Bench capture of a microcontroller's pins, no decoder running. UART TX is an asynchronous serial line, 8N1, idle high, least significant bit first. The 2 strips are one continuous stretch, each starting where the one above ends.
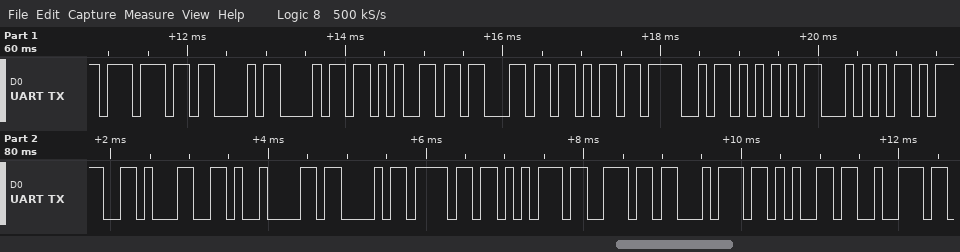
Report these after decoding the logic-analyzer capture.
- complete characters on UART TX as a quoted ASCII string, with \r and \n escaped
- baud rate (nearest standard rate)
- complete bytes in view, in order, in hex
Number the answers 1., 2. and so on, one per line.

1. "wCheckOUT=1\tCounter"
2. 9600 baud
3. 77 43 68 65 63 6B 4F 55 54 3D 31 09 43 6F 75 6E 74 65 72
